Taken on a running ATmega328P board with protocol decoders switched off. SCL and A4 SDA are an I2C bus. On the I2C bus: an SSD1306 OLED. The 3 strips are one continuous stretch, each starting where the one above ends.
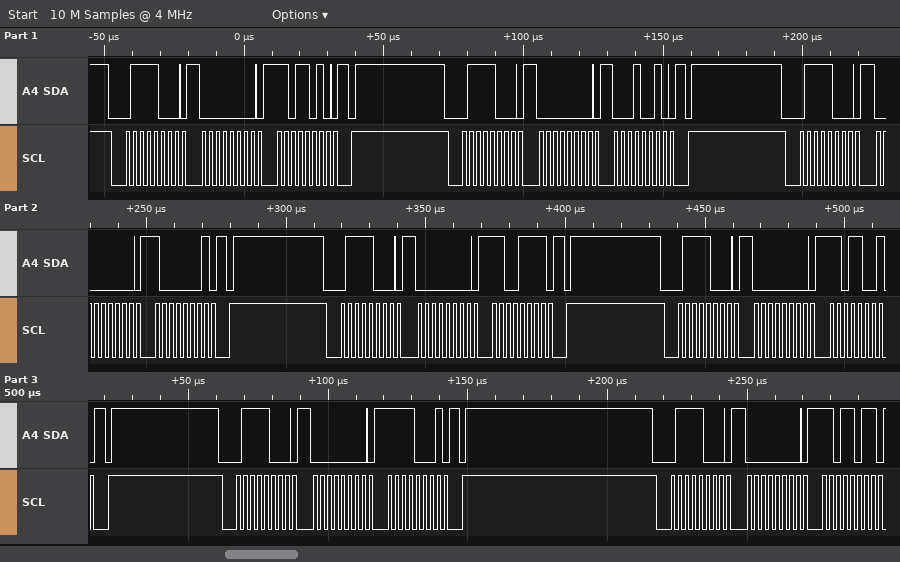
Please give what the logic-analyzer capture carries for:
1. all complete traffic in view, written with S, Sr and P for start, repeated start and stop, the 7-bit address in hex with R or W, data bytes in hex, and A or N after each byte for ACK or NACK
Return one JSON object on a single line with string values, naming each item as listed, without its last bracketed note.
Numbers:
{"all complete traffic in view, written with S, Sr and P for start, repeated start and stop, the 7-bit address in hex with R or W, data bytes in hex, and A or N after each byte for ACK or NACK": "S 3CW A 00 A DA A P S 3CW A 00 A 12 A P S 3CW A 00 A 81 A P S 3CW A 00 A CF A P S 3CW A 00 A D9 A P S 3CW A 00 A F1 A P S 3CW A 00 A DB A"}
